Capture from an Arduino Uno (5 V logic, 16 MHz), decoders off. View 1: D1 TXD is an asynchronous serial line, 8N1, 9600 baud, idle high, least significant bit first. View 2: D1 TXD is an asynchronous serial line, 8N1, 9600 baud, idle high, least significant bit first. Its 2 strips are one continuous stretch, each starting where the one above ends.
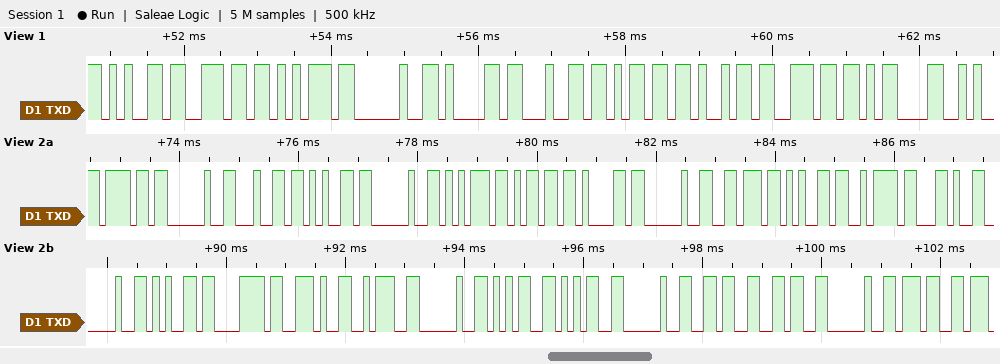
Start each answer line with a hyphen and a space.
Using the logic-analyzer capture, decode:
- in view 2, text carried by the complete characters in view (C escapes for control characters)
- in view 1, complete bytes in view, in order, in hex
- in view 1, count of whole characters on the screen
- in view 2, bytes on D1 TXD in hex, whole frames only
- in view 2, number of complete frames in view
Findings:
- "o de uma vez, ex.: 55 66 7"
- 65 6E 75 20 61 64 6D 69 6E 0D
- 10
- 6F 20 64 65 20 75 6D 61 20 76 65 7A 2C 20 65 78 2E 3A 20 35 35 20 36 36 20 37
- 26
